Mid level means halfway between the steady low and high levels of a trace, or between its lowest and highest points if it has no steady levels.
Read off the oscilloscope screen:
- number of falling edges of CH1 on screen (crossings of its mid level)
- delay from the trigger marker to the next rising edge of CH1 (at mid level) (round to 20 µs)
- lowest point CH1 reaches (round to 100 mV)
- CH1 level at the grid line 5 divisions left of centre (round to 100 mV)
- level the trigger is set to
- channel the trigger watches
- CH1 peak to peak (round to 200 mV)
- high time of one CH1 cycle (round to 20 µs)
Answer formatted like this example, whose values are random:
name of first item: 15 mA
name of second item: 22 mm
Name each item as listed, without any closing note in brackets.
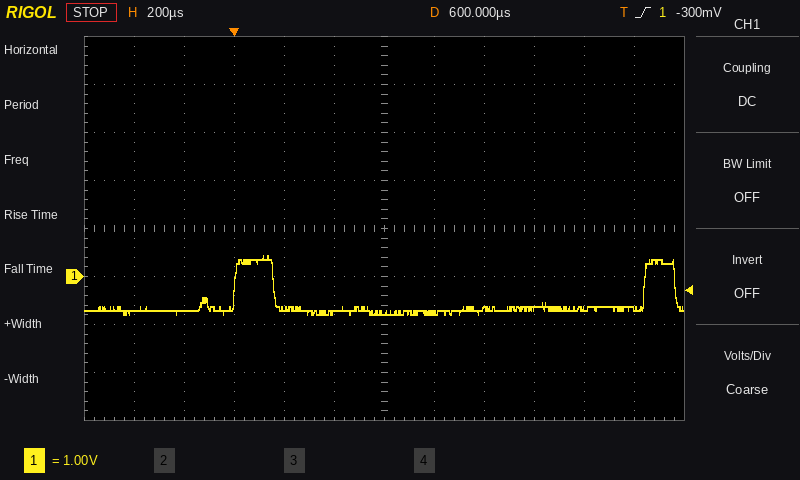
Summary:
number of falling edges of CH1 on screen: 2
delay from the trigger marker to the next rising edge of CH1 (at mid level): 1.64 ms
lowest point CH1 reaches: -800 mV
CH1 level at the grid line 5 divisions left of centre: -700 mV
level the trigger is set to: -300 mV
channel the trigger watches: CH1
CH1 peak to peak: 1.2 V
high time of one CH1 cycle: 140 µs
